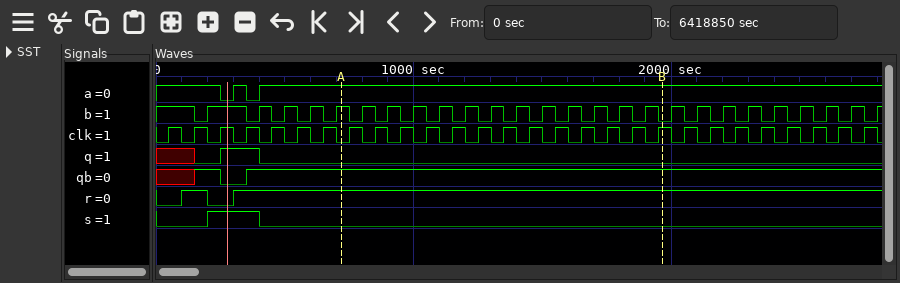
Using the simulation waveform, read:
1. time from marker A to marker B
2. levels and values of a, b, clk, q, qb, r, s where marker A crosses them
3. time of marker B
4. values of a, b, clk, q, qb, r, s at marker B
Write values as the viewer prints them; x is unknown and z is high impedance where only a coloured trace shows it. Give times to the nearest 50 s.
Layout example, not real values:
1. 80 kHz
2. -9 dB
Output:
1. 1250 s
2. a=1, b=1, clk=0, q=0, qb=1, r=1, s=0
3. 1950 s
4. a=1, b=0, clk=1, q=0, qb=1, r=1, s=0
